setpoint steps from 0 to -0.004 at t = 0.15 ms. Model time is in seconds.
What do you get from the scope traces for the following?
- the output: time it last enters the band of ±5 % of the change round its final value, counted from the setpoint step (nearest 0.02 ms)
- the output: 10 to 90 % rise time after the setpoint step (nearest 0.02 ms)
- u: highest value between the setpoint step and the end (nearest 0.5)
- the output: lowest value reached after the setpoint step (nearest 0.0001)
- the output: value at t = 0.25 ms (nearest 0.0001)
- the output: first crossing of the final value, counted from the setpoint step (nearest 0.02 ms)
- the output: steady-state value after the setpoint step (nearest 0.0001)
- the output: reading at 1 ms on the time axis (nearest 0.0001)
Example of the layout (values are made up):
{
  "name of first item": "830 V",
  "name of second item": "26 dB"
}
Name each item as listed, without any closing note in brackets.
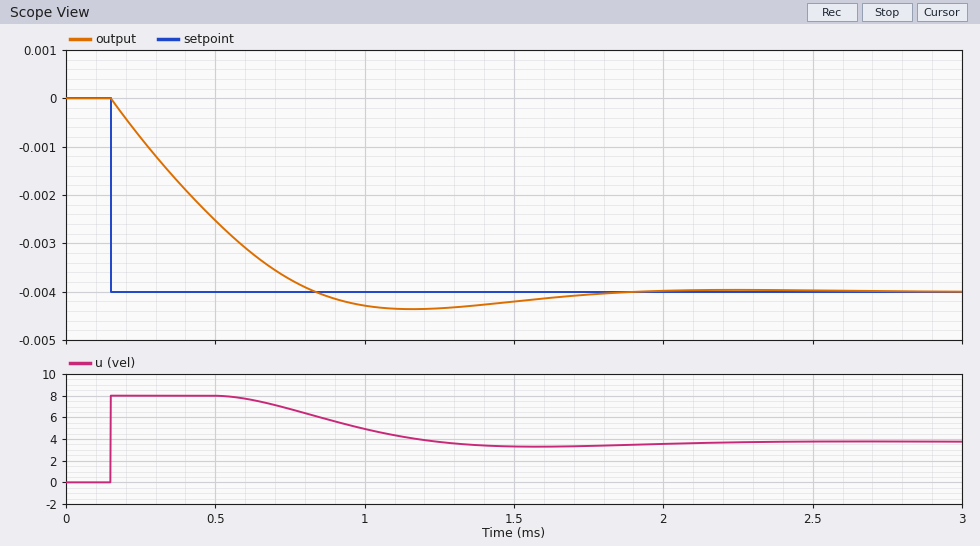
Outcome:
{
  "the output: time it last enters the band of ±5 % of the change round its final value, counted from the setpoint step": "1.36 ms",
  "the output: 10 to 90 % rise time after the setpoint step": "0.52 ms",
  "u: highest value between the setpoint step and the end": "8.0",
  "the output: lowest value reached after the setpoint step": "-0.0044",
  "the output: value at t = 0.25 ms": "-0.0008",
  "the output: first crossing of the final value, counted from the setpoint step": "0.68 ms",
  "the output: steady-state value after the setpoint step": "-0.0040",
  "the output: reading at 1 ms on the time axis": "-0.0043"
}
